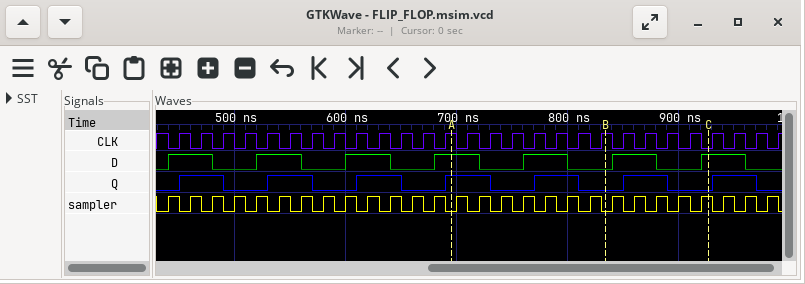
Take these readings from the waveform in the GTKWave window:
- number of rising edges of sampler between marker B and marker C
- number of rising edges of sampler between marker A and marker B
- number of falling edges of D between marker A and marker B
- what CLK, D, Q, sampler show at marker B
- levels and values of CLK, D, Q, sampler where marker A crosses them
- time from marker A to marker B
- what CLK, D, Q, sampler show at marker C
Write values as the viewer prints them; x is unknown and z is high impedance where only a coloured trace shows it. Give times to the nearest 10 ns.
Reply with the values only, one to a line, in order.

5
7
2
CLK=1, D=0, Q=0, sampler=0
CLK=1, D=1, Q=1, sampler=0
140 ns
CLK=0, D=1, Q=0, sampler=1
